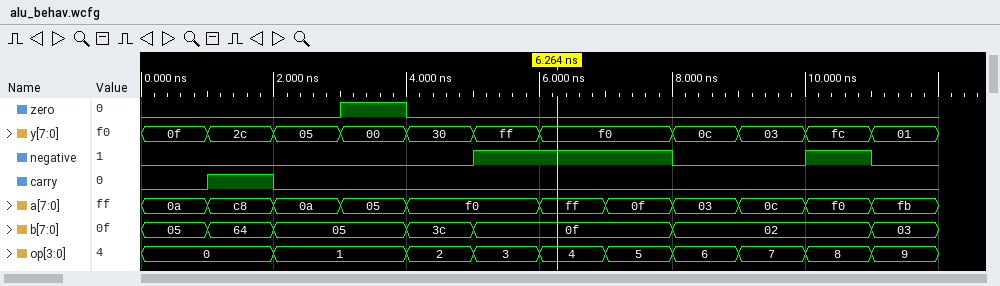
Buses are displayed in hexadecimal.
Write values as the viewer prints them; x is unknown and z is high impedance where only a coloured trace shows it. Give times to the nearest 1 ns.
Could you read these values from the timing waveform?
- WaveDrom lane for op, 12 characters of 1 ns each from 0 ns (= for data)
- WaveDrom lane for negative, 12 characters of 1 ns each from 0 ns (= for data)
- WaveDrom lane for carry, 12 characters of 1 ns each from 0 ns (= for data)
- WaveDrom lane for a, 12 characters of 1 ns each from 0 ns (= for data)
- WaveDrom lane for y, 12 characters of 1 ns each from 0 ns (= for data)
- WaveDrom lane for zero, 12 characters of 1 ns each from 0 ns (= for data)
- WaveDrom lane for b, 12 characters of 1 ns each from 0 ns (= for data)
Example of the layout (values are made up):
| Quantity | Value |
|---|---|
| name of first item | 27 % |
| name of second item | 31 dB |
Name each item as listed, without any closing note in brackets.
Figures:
| Quantity | Value |
|---|---|
| WaveDrom lane for op, 12 characters of 1 ns each from 0 ns | {name: 'op', wave: '=.=.========', data: '0 1 2 3 4 5 6 7 8 9'} |
| WaveDrom lane for negative, 12 characters of 1 ns each from 0 ns | {name: 'negative', wave: '0....1..0.10'} |
| WaveDrom lane for carry, 12 characters of 1 ns each from 0 ns | {name: 'carry', wave: '010.........'} |
| WaveDrom lane for a, 12 characters of 1 ns each from 0 ns | {name: 'a', wave: '=====.======', data: '0a c8 0a 05 f0 ff 0f 03 0c f0 fb'} |
| WaveDrom lane for y, 12 characters of 1 ns each from 0 ns | {name: 'y', wave: '=======.====', data: '0f 2c 05 00 30 ff f0 0c 03 fc 01'} |
| WaveDrom lane for zero, 12 characters of 1 ns each from 0 ns | {name: 'zero', wave: '0..10.......'} |
| WaveDrom lane for b, 12 characters of 1 ns each from 0 ns | {name: 'b', wave: '===.==..=..=', data: '05 64 05 3c 0f 02 03'} |
